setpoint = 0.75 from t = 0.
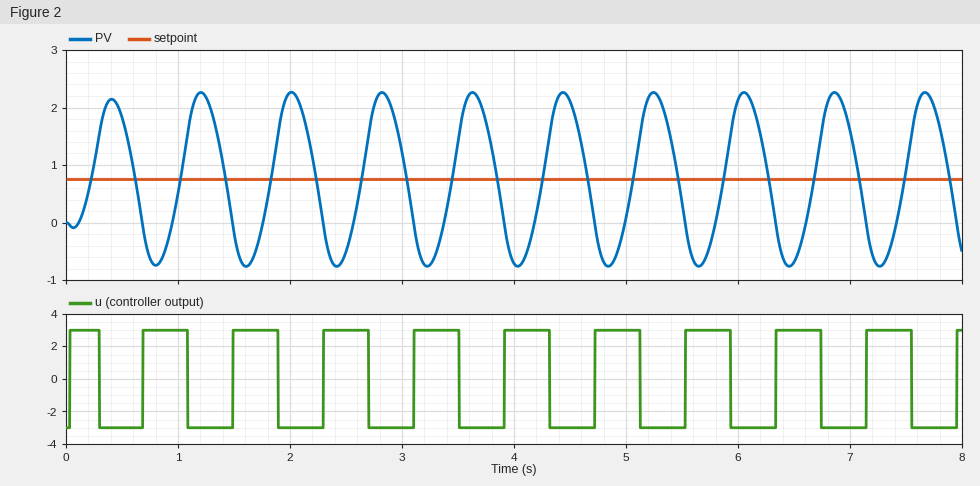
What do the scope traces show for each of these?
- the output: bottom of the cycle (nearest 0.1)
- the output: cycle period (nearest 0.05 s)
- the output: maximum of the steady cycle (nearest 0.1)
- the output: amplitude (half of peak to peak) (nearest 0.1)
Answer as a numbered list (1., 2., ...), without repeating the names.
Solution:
1. -0.8
2. 0.80 s
3. 2.3
4. 1.5
